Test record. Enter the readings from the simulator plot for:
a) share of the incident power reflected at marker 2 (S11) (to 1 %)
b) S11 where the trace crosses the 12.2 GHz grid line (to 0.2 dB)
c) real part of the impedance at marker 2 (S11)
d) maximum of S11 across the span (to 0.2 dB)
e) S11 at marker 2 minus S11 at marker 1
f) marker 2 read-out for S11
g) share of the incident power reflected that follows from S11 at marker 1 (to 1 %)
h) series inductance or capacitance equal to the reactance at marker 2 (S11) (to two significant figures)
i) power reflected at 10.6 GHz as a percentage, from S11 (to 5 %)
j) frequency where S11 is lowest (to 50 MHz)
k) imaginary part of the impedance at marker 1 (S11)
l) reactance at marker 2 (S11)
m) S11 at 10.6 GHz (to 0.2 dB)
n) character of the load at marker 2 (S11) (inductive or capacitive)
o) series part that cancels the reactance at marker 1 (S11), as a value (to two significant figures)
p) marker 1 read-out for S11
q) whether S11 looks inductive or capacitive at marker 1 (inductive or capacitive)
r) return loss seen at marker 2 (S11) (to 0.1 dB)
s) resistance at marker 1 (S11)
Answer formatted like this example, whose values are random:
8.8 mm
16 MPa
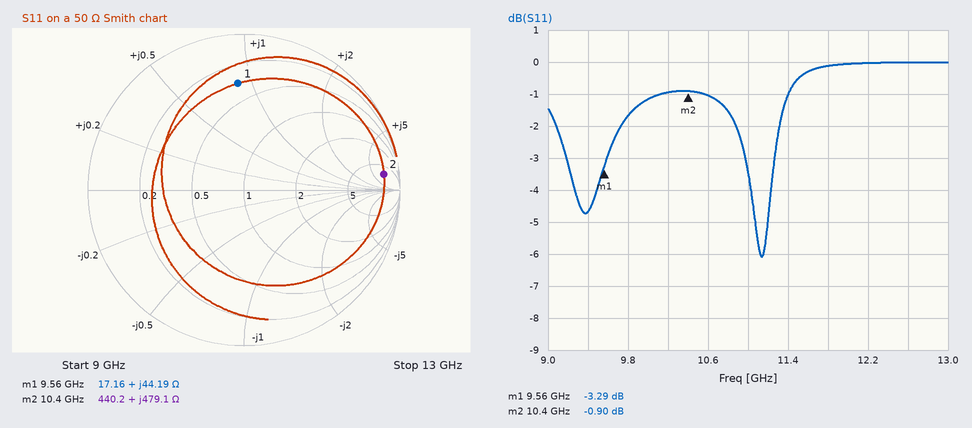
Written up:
81 %
0.0 dB
440.2 Ω
0.0 dB
2.39 dB
-0.90 dB
47 %
7.3 nH
80 %
11.15 GHz
+44.19 Ω
+479.1 Ω
-1.0 dB
inductive
380 fF
-3.29 dB
inductive
0.9 dB
17.16 Ω
